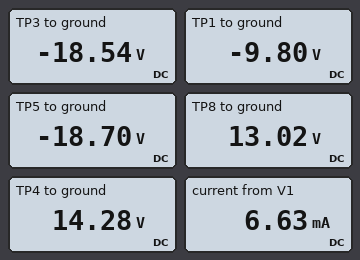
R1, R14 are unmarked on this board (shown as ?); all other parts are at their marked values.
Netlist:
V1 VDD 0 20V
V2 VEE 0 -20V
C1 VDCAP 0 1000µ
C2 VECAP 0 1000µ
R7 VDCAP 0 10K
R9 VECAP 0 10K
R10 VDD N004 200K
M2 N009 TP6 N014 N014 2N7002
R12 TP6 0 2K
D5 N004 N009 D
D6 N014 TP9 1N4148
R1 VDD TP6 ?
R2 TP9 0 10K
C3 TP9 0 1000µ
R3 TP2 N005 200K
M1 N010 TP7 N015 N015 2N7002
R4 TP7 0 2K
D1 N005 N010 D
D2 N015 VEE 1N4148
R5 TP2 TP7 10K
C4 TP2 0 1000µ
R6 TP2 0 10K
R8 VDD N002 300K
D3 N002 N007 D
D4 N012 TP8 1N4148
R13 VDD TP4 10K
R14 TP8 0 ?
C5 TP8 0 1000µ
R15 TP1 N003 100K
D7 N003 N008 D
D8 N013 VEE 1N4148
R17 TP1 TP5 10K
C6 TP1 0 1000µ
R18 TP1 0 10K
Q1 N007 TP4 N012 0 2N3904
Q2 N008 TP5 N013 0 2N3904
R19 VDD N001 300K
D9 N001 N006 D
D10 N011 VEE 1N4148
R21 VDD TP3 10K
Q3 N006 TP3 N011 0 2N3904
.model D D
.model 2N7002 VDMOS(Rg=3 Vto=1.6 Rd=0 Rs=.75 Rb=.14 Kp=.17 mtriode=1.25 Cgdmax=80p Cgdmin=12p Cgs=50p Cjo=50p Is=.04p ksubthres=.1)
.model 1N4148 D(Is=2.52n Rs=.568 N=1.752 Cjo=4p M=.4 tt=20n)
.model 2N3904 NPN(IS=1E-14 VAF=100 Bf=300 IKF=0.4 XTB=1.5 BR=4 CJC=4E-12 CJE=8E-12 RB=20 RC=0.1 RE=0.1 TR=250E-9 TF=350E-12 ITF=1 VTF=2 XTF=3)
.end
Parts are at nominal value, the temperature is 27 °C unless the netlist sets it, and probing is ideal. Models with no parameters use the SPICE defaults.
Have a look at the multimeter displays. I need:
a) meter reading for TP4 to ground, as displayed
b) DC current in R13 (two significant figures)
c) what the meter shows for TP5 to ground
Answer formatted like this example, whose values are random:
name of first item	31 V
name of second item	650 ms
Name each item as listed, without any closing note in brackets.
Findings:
meter reading for TP4 to ground, as displayed	14.28 V
DC current in R13	570 µA
what the meter shows for TP5 to ground	-18.70 V
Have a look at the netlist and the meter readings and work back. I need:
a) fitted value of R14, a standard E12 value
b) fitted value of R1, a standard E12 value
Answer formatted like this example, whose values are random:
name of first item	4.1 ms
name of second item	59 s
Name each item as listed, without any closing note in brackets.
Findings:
fitted value of R14, a standard E12 value	22 kΩ
fitted value of R1, a standard E12 value	8.2 kΩ
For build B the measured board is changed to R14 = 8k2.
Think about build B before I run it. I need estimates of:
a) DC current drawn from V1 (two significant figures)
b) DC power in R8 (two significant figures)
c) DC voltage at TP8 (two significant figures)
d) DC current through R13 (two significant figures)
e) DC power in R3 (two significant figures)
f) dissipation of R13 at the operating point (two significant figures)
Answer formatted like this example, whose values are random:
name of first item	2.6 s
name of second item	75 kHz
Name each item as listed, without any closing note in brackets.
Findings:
DC current drawn from V1	7.1 mA
DC power in R8	350 µW
DC voltage at TP8	8.6 V
DC current through R13	1.0 mA
DC power in R3	1.7 mW
dissipation of R13 at the operating point	10 mW
